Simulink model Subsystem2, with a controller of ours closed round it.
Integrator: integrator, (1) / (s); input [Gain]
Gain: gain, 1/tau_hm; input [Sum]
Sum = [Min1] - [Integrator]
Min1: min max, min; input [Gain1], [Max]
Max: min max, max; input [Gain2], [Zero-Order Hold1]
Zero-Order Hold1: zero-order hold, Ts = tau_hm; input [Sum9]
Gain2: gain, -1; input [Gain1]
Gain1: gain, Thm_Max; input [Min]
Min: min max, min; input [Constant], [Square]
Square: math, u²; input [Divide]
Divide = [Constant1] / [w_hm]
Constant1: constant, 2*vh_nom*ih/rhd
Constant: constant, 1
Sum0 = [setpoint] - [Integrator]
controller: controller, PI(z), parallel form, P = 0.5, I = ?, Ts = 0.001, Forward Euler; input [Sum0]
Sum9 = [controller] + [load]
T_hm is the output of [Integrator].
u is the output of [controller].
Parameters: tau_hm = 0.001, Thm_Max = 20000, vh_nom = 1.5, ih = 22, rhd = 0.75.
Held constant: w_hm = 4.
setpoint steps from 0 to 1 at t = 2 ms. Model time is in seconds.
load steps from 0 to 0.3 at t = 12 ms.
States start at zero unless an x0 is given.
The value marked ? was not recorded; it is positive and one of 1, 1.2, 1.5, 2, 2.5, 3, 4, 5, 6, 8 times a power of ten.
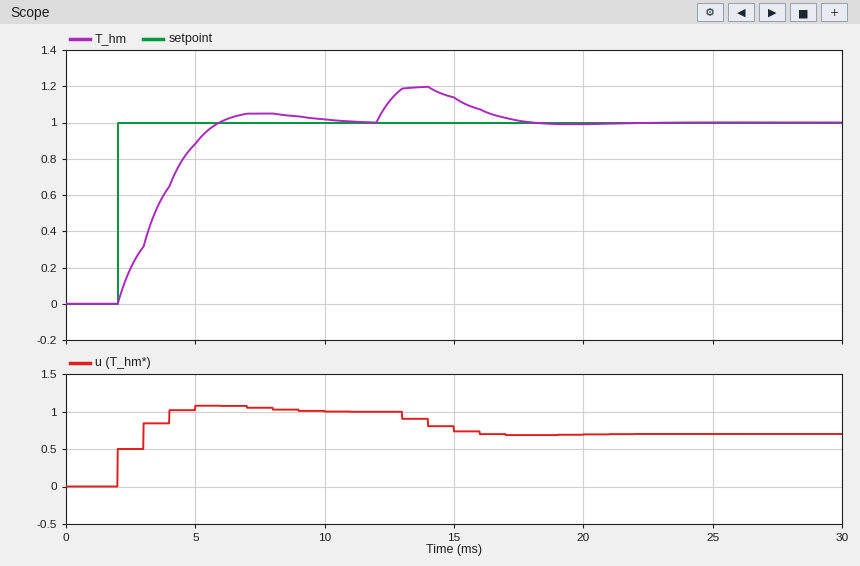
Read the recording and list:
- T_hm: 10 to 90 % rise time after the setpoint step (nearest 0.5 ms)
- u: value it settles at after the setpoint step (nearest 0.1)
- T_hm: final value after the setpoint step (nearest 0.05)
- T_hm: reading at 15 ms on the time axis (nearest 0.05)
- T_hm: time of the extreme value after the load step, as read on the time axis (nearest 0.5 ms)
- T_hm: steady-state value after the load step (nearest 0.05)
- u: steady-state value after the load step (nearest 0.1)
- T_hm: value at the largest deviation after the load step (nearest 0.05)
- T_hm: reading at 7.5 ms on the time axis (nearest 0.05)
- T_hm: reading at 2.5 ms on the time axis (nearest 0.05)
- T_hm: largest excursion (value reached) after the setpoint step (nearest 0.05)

3.0 ms
1.0
1.00
1.15
14.0 ms
1.00
0.7
1.20
1.05
0.20
1.05
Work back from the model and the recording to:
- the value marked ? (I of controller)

500
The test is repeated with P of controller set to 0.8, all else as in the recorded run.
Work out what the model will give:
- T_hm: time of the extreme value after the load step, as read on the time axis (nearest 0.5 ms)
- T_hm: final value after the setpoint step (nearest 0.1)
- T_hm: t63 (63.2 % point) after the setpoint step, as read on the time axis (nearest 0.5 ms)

13.0 ms
1.0
3.5 ms
